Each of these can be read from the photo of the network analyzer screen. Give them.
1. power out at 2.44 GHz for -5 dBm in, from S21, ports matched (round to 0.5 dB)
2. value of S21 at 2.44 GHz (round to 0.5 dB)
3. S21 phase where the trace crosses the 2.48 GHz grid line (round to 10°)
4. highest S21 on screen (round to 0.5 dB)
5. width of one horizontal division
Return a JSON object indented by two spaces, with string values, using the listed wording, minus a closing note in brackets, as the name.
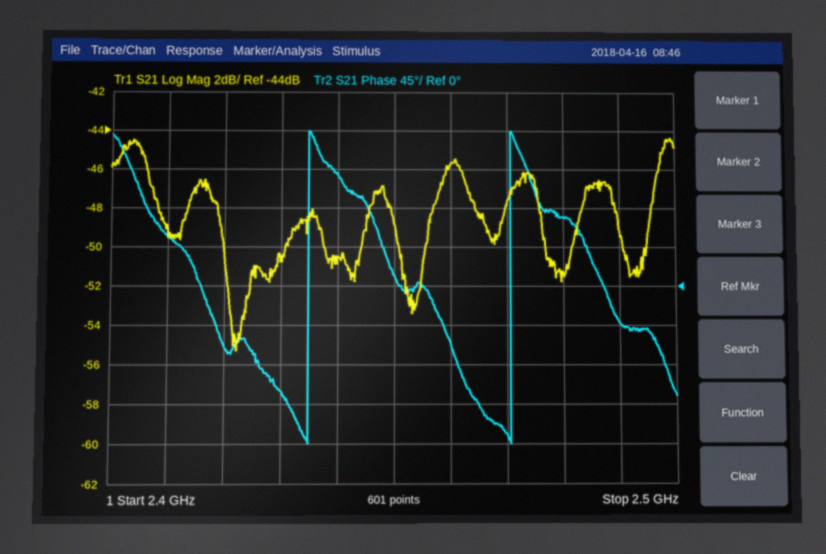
{
  "power out at 2.44 GHz for -5 dBm in, from S21, ports matched": "-55.5 dBm",
  "value of S21 at 2.44 GHz": "-50.5 dB",
  "S21 phase where the trace crosses the 2.48 GHz grid line": "80°",
  "highest S21 on screen": "-44.5 dB",
  "width of one horizontal division": "10 MHz"
}
